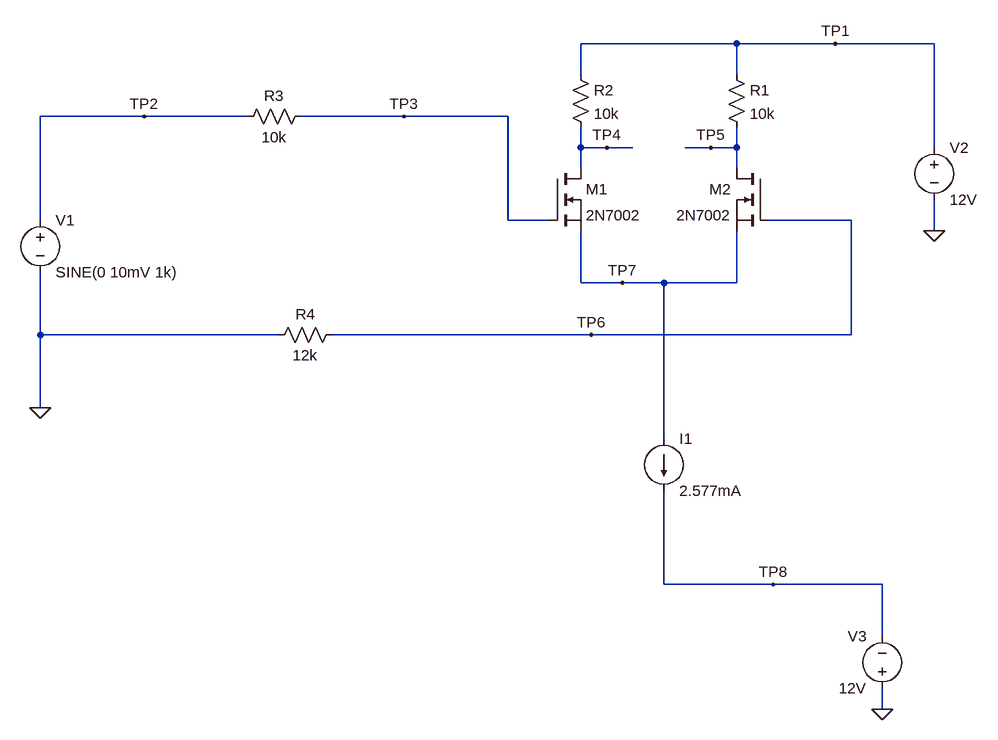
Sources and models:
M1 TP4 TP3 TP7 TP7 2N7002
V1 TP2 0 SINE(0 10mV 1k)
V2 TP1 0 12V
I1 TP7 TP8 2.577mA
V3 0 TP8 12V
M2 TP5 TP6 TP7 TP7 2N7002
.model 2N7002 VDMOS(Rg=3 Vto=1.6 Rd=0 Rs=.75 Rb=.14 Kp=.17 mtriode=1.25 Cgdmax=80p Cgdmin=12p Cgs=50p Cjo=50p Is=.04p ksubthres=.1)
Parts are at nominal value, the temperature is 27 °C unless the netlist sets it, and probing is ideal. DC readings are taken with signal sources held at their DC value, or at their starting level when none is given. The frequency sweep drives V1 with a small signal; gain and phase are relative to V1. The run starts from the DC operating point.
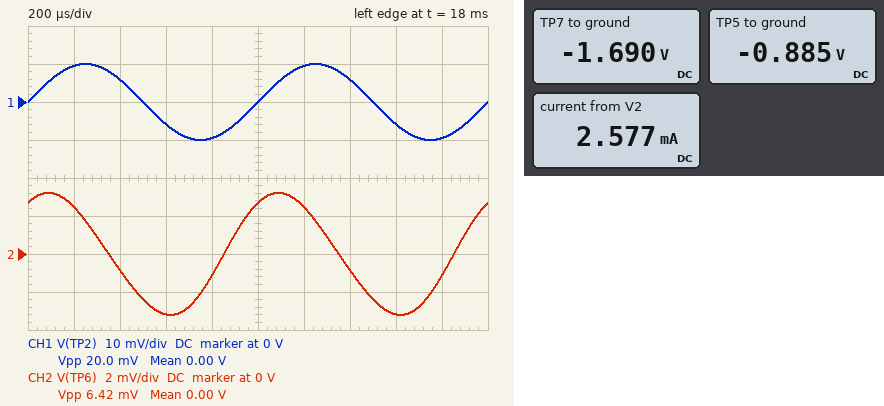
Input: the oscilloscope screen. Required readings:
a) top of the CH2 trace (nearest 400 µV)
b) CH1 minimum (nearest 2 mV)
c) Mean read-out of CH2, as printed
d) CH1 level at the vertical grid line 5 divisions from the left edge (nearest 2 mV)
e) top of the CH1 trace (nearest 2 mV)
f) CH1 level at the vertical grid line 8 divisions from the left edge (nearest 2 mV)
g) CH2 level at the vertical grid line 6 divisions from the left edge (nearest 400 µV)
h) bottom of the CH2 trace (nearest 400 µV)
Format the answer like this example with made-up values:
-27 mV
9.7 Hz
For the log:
3.2 mV
-10 mV
0.00 V
0 V
10 mV
-6 mV
2.4 mV
-3.2 mV
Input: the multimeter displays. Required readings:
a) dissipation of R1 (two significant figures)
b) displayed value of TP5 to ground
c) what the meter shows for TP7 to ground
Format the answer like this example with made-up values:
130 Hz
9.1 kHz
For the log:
17 mW
-0.885 V
-1.690 V
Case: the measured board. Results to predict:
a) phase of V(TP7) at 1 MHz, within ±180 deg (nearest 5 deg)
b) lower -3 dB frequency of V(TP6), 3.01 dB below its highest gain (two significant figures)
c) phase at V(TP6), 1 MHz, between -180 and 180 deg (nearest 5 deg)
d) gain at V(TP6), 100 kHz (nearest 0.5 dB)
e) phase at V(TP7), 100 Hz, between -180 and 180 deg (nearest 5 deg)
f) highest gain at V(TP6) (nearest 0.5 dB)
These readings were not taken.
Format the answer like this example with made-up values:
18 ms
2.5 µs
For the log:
-5 deg
1.3 kHz
-5 deg
-7.5 dB
0 deg
-5.5 dB
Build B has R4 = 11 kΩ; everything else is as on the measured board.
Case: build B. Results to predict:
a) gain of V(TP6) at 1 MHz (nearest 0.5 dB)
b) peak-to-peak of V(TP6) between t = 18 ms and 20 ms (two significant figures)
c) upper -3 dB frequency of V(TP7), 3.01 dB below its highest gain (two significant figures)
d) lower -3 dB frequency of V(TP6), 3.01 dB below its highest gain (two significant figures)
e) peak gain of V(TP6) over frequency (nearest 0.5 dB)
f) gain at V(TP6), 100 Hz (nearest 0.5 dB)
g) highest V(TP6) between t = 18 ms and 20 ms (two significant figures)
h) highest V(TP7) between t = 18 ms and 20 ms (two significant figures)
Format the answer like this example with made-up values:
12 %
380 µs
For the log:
-12.0 dB
6.0 mV
150 kHz
1.4 kHz
-6.0 dB
-28.5 dB
3.0 mV
-1.7 V
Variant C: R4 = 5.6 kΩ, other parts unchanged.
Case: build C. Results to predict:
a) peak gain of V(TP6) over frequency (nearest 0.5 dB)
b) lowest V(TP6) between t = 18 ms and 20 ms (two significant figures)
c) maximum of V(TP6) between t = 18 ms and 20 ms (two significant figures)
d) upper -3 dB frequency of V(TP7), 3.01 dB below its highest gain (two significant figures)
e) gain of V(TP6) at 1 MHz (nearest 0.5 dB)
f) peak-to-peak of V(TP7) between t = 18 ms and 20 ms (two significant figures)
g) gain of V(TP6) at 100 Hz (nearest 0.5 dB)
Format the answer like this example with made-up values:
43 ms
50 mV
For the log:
-9.0 dB
-1.7 mV
1.6 mV
33 kHz
-13.5 dB
9.5 mV
-34.5 dB
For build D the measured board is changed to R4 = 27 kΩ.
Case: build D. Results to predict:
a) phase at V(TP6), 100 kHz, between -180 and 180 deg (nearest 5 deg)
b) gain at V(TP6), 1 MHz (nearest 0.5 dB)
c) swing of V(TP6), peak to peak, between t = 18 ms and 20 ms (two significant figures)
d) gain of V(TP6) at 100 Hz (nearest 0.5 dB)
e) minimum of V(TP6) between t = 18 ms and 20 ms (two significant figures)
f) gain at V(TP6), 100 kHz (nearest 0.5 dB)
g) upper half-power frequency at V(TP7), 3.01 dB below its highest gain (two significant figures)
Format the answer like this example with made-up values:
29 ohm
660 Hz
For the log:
-25 deg
-10.5 dB
11 mV
-21.0 dB
-5.6 mV
-5.5 dB
110 kHz
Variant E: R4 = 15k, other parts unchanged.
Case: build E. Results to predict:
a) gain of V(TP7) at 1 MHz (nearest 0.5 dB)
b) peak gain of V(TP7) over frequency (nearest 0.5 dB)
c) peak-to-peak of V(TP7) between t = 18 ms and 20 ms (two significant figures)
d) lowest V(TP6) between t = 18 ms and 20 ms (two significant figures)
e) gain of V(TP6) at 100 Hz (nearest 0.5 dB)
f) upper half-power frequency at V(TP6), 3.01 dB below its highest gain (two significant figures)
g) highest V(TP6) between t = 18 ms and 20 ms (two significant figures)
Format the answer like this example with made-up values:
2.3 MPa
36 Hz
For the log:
-11.0 dB
-4.5 dB
11 mV
-3.8 mV
-26.0 dB
130 kHz
3.8 mV
